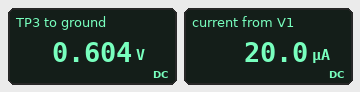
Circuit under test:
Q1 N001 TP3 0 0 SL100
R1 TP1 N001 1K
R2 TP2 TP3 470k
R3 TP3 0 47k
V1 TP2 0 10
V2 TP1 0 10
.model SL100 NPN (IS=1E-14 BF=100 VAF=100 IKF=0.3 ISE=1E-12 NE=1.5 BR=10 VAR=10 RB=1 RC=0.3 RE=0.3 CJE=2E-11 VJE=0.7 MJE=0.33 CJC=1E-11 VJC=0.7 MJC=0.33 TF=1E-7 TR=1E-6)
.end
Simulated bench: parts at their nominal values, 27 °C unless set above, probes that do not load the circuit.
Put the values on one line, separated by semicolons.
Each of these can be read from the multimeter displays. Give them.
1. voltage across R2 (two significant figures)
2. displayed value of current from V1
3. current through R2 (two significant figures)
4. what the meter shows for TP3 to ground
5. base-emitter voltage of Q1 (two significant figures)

9.4 V; 20.0 µA; 20 µA; 0.604 V; 600 mV
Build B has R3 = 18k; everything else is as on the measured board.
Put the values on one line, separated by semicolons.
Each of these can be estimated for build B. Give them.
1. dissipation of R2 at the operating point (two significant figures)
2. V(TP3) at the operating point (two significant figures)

200 µW; 370 mV
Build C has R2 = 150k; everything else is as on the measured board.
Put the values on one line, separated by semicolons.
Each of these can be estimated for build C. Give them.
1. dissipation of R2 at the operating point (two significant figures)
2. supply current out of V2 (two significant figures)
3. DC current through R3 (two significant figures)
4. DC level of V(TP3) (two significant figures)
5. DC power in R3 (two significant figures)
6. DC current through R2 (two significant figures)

580 µW; 1.7 mA; 14 µA; 670 mV; 9.5 µW; 62 µA
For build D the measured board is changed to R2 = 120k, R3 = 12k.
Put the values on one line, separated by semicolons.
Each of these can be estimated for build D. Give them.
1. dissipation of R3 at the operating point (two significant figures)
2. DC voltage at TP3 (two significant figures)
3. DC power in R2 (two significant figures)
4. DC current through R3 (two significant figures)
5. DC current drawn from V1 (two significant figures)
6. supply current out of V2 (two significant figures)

35 µW; 650 mV; 730 µW; 54 µA; 78 µA; 720 µA
